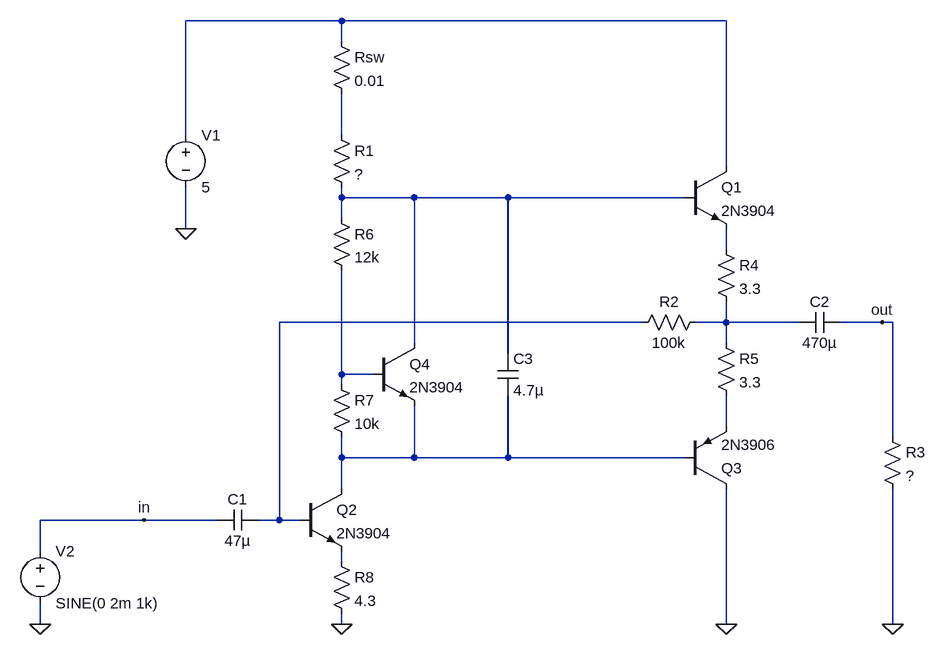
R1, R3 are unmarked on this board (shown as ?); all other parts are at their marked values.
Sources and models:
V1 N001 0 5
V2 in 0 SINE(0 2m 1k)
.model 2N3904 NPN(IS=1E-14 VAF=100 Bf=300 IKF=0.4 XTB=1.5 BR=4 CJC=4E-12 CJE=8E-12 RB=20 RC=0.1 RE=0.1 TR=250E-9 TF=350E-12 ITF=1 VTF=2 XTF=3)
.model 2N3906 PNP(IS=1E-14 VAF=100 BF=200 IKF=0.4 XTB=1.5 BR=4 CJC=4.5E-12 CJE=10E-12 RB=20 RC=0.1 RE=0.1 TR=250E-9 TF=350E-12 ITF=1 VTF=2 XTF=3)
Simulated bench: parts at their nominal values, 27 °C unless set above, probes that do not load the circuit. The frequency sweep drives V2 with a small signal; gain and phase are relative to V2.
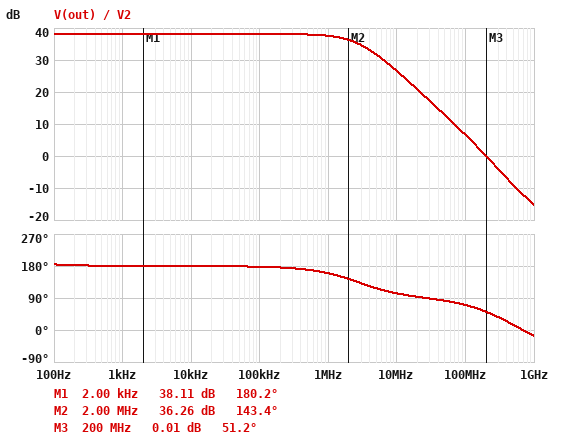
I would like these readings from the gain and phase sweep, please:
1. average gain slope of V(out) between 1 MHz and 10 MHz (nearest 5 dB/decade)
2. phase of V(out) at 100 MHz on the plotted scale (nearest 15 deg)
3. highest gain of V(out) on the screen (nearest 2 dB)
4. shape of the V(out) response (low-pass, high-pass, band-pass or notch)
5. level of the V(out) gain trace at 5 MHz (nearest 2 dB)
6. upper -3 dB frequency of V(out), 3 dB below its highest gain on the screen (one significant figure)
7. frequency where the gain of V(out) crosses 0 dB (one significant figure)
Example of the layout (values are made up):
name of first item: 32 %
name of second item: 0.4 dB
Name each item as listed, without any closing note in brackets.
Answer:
average gain slope of V(out) between 1 MHz and 10 MHz: -10 dB/decade
phase of V(out) at 100 MHz on the plotted scale: 75 deg
highest gain of V(out) on the screen: 38 dB
shape of the V(out) response: low-pass
level of the V(out) gain trace at 5 MHz: 32 dB
upper -3 dB frequency of V(out), 3 dB below its highest gain on the screen: 3 MHz
frequency where the gain of V(out) crosses 0 dB: 200 MHz
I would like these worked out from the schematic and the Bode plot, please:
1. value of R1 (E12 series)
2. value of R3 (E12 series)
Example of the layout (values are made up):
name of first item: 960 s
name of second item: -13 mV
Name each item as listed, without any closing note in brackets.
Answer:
value of R1: 3.3 kΩ
value of R3: 56 Ω
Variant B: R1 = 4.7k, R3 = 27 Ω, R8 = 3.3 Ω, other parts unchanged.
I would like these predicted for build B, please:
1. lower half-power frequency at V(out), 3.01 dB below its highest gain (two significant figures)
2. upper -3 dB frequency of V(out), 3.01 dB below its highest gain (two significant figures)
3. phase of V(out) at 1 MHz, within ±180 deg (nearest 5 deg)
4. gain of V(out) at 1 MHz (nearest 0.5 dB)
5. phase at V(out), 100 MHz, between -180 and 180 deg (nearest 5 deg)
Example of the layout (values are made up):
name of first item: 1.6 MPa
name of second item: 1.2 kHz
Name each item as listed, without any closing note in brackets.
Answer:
lower half-power frequency at V(out), 3.01 dB below its highest gain: 7.7 Hz
upper -3 dB frequency of V(out), 3.01 dB below its highest gain: 1.7 MHz
phase of V(out) at 1 MHz, within ±180 deg: 150 deg
gain of V(out) at 1 MHz: 34.0 dB
phase at V(out), 100 MHz, between -180 and 180 deg: 60 deg
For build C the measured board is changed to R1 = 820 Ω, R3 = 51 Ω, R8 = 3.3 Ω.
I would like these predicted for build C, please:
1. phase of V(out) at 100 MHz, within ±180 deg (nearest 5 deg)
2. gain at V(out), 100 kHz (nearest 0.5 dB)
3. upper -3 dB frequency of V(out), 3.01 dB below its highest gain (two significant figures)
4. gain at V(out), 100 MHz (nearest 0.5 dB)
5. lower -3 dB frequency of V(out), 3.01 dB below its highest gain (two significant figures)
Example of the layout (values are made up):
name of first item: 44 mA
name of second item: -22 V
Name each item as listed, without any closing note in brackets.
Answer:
phase of V(out) at 100 MHz, within ±180 deg: 75 deg
gain at V(out), 100 kHz: 35.5 dB
upper -3 dB frequency of V(out), 3.01 dB below its highest gain: 8.7 MHz
gain at V(out), 100 MHz: 14.0 dB
lower -3 dB frequency of V(out), 3.01 dB below its highest gain: 7.0 Hz
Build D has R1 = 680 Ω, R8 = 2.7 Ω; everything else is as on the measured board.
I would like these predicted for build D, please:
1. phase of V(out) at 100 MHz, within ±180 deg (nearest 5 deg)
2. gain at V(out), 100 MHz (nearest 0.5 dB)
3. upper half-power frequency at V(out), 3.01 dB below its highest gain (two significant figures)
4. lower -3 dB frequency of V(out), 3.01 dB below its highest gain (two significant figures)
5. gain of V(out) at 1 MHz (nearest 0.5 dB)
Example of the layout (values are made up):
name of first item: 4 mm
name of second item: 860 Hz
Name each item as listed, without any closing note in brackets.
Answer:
phase of V(out) at 100 MHz, within ±180 deg: 75 deg
gain at V(out), 100 MHz: 15.0 dB
upper half-power frequency at V(out), 3.01 dB below its highest gain: 10 MHz
lower -3 dB frequency of V(out), 3.01 dB below its highest gain: 6.7 Hz
gain of V(out) at 1 MHz: 35.5 dB
